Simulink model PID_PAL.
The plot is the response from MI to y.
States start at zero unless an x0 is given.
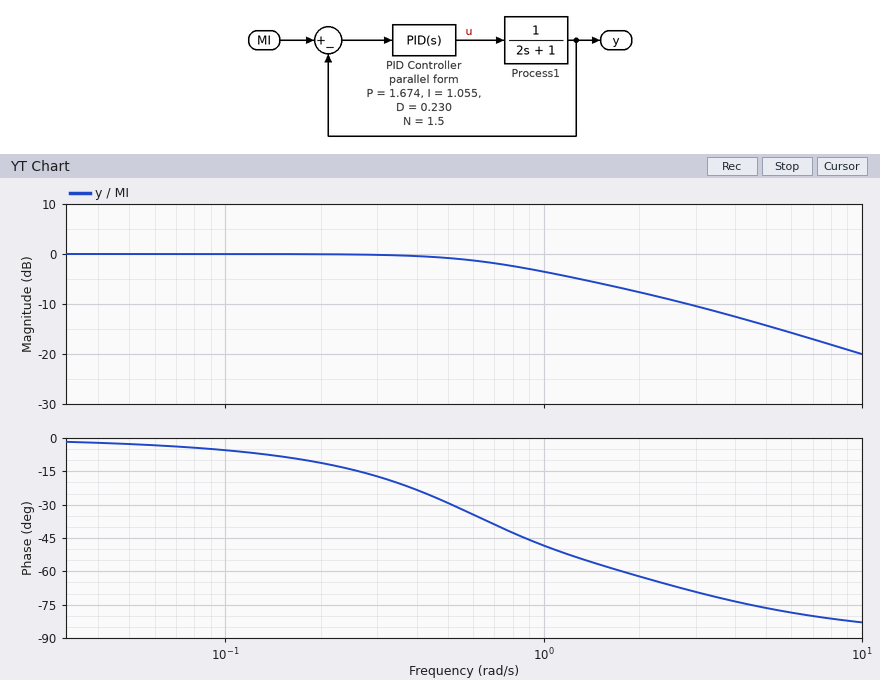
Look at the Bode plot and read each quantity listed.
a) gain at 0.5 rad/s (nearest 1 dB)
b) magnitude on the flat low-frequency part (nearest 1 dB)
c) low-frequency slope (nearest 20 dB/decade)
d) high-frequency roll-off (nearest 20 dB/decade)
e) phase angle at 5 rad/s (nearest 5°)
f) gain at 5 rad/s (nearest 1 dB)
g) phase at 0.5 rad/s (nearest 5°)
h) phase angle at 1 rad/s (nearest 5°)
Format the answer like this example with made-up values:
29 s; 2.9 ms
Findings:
-1 dB; 0 dB; 0 dB/decade; -20 dB/decade; -75°; -14 dB; -30°; -50°
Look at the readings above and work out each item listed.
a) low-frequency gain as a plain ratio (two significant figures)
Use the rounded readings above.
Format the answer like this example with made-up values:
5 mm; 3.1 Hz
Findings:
1.0
